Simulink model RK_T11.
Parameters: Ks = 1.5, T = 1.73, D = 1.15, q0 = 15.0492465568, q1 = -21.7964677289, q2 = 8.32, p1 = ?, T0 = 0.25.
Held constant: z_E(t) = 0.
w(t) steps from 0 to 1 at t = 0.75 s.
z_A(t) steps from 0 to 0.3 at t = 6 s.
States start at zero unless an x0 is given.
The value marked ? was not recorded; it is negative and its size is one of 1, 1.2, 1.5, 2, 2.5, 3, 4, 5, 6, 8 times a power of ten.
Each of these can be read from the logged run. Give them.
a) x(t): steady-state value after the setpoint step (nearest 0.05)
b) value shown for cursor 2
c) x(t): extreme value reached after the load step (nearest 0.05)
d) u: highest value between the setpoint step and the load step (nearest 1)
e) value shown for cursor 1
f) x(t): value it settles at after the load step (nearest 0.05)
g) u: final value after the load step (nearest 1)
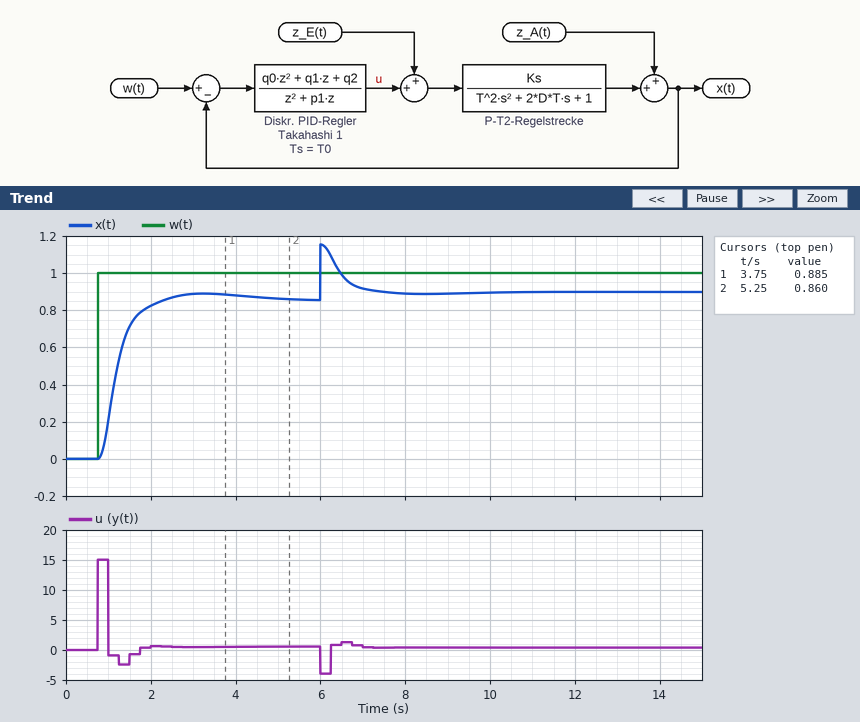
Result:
0.85
0.860
1.15
15
0.885
0.90
0
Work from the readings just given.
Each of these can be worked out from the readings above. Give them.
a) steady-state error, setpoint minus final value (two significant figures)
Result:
0.15
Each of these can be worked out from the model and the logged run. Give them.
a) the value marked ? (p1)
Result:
-0.6
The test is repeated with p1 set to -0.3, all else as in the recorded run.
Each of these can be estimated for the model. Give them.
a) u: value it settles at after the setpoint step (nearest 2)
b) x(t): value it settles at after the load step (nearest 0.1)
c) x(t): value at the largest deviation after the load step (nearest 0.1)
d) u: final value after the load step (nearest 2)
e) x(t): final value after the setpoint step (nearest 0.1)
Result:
0
0.8
1.1
0
0.8
